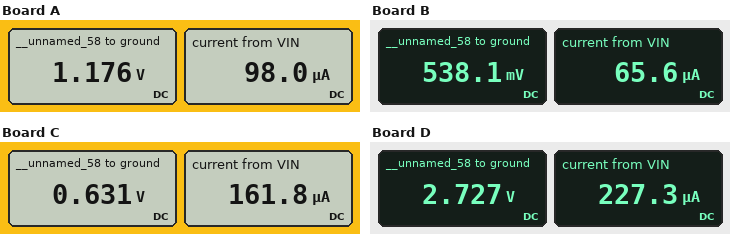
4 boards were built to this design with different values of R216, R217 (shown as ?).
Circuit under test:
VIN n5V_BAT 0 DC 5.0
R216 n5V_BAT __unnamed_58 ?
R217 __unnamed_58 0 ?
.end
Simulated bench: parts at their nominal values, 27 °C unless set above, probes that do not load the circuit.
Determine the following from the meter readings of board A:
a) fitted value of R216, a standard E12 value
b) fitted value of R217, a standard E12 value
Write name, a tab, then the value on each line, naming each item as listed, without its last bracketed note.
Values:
fitted value of R216, a standard E12 value	39 kΩ
fitted value of R217, a standard E12 value	12 kΩ
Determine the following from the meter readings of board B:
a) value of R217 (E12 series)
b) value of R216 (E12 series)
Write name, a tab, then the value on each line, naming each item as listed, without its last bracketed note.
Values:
value of R217	8.2 kΩ
value of R216	68 kΩ
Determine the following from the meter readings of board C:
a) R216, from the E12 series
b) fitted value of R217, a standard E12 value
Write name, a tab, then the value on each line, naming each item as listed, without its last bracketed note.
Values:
R216, from the E12 series	27 kΩ
fitted value of R217, a standard E12 value	3.9 kΩ
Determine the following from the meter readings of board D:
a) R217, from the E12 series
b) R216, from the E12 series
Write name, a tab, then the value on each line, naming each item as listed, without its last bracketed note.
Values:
R217, from the E12 series	12 kΩ
R216, from the E12 series	10 kΩ
